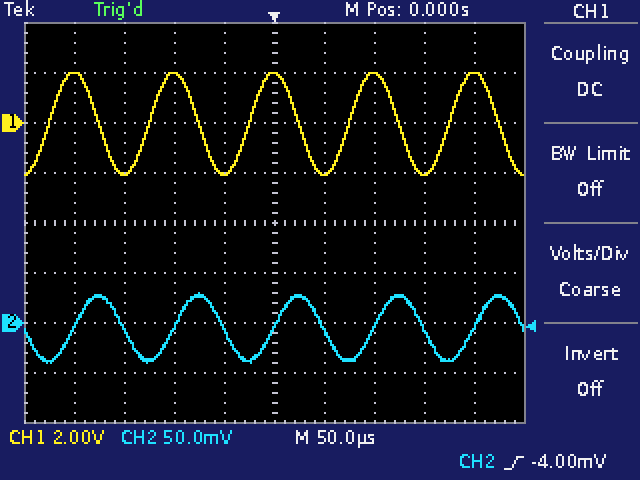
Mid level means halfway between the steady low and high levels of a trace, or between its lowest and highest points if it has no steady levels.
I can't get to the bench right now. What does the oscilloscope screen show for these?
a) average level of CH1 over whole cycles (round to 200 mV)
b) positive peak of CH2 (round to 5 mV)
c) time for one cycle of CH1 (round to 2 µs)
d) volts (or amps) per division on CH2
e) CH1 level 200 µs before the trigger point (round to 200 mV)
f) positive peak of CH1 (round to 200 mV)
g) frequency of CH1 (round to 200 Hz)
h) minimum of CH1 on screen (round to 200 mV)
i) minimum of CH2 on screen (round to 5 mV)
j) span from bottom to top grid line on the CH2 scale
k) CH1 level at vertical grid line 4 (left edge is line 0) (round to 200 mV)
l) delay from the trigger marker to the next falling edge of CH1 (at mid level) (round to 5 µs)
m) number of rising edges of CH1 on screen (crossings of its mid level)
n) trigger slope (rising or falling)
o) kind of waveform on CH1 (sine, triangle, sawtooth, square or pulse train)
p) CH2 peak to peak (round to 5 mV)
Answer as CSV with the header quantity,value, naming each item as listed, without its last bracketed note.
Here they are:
quantity,value
average level of CH1 over whole cycles,0.0 V
positive peak of CH2,30 mV
time for one cycle of CH1,100 µs
volts (or amps) per division on CH2,50 mV
CH1 level 200 µs before the trigger point,2.0 V
positive peak of CH1,2.0 V
frequency of CH1,10.0 kHz
minimum of CH1 on screen,-2.0 V
minimum of CH2 on screen,-40 mV
span from bottom to top grid line on the CH2 scale,400 mV
CH1 level at vertical grid line 4 (left edge is line 0),-2.0 V
delay from the trigger marker to the next falling edge of CH1 (at mid level),25 µs
number of rising edges of CH1 on screen,5
trigger slope,rising
kind of waveform on CH1,sine
CH2 peak to peak,70 mV
